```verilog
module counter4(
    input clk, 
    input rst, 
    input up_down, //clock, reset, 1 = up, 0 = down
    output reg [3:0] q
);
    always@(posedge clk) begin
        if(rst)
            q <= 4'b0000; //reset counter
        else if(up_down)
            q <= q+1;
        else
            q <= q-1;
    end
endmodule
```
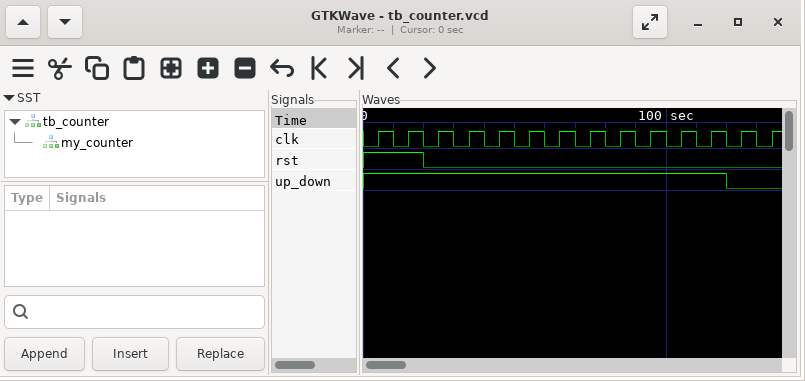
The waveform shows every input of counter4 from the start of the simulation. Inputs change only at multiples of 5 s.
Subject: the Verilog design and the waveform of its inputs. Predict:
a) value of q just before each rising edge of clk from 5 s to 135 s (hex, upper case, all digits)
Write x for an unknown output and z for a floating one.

x, 0, 0, 1, 2, 3, 4, 5, 6, 7, 8, 9, A, 9
